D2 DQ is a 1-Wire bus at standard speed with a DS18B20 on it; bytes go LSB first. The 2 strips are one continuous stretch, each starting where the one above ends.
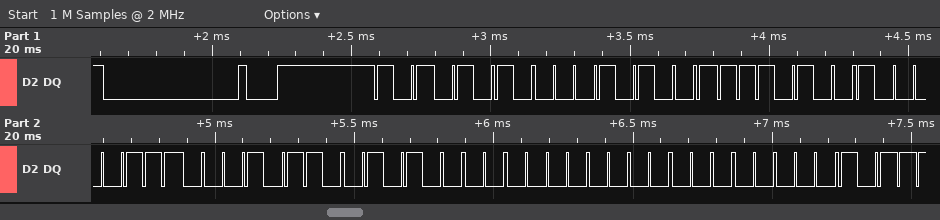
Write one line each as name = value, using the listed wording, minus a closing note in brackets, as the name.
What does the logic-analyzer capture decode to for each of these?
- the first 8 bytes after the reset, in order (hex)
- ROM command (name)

the first 8 bytes after the reset, in order = 55 28 2F E1 68 0A 00 00
ROM command = Match ROM
